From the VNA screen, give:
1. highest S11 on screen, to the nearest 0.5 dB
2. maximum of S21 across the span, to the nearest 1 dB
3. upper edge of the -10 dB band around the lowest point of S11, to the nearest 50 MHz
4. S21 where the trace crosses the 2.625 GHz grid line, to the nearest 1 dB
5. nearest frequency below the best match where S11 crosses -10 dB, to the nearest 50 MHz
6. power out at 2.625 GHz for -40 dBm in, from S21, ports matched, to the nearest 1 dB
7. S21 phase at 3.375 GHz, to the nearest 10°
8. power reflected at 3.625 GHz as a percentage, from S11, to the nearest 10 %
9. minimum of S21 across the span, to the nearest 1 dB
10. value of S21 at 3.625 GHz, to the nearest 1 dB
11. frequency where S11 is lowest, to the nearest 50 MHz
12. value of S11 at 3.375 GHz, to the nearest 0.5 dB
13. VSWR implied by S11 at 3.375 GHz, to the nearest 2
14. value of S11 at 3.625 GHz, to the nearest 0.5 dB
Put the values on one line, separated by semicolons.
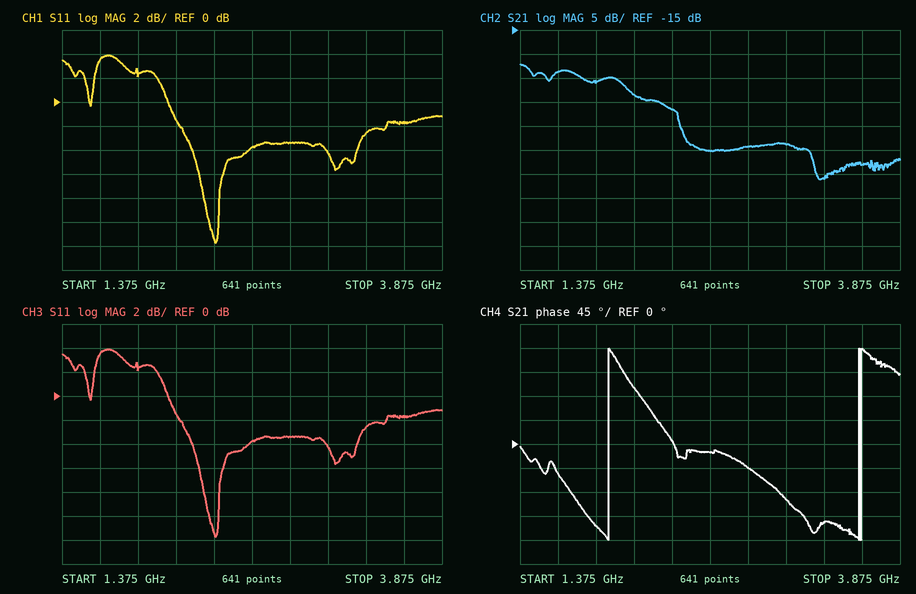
4.0 dB; -22 dB; 2.40 GHz; -40 dB; 2.35 GHz; -80 dBm; -150°; 70 %; -46 dB; -43 dB; 2.40 GHz; -2.5 dB; 6; -1.5 dB
